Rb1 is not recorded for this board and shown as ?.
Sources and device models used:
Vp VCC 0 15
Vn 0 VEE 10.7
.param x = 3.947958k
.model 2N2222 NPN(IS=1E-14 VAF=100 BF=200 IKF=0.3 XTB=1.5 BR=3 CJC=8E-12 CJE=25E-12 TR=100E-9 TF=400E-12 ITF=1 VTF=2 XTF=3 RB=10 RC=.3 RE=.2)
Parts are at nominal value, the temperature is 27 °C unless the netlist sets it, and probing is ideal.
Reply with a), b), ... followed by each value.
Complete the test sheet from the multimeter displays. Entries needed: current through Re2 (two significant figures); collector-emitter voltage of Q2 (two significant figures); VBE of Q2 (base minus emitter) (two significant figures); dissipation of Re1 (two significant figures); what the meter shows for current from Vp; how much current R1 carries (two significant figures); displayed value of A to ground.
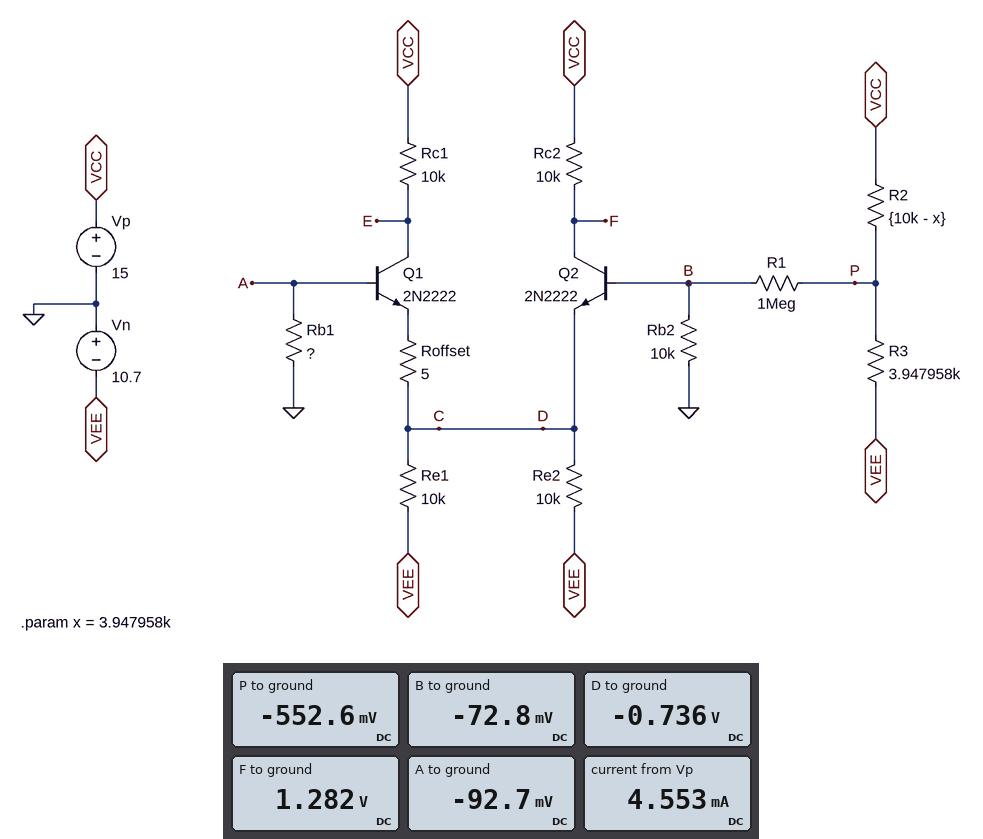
a) 1.0 mA
b) 2.0 V
c) 660 mV
d) 9.9 mW
e) 4.553 mA
f) 480 nA
g) -92.7 mV
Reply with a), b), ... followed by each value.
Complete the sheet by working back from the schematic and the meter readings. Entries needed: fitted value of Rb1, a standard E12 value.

a) 33 kΩ
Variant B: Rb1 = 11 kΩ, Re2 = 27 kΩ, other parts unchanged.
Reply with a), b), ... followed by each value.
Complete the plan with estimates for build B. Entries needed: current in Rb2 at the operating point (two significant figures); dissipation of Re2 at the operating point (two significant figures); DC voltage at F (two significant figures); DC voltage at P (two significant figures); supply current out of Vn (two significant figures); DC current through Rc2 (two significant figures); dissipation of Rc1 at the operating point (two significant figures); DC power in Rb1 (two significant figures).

a) 3.7 µA
b) 3.7 mW
c) 8.1 V
d) -550 mV
e) 3.9 mA
f) 690 µA
g) 4.6 mW
h) 110 nW
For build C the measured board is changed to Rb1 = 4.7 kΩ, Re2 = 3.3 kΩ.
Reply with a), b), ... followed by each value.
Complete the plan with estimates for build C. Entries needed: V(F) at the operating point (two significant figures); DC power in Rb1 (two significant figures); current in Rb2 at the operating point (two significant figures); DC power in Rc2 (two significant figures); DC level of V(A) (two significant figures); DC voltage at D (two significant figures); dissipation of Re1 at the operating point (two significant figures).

a) -1.6 V
b) 210 µW
c) 100 µA
d) 28 mW
e) -990 mV
f) -1.7 V
g) 8.1 mW
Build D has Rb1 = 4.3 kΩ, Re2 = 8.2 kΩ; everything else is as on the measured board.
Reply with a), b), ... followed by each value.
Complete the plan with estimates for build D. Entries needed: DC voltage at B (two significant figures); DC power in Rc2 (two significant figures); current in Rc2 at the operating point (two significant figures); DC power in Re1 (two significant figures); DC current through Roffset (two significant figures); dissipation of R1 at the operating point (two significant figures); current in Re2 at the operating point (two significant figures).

a) -47 mV
b) 7.8 mW
c) 880 µA
d) 10 mW
e) 1.3 mA
f) 260 nW
g) 1.2 mA
